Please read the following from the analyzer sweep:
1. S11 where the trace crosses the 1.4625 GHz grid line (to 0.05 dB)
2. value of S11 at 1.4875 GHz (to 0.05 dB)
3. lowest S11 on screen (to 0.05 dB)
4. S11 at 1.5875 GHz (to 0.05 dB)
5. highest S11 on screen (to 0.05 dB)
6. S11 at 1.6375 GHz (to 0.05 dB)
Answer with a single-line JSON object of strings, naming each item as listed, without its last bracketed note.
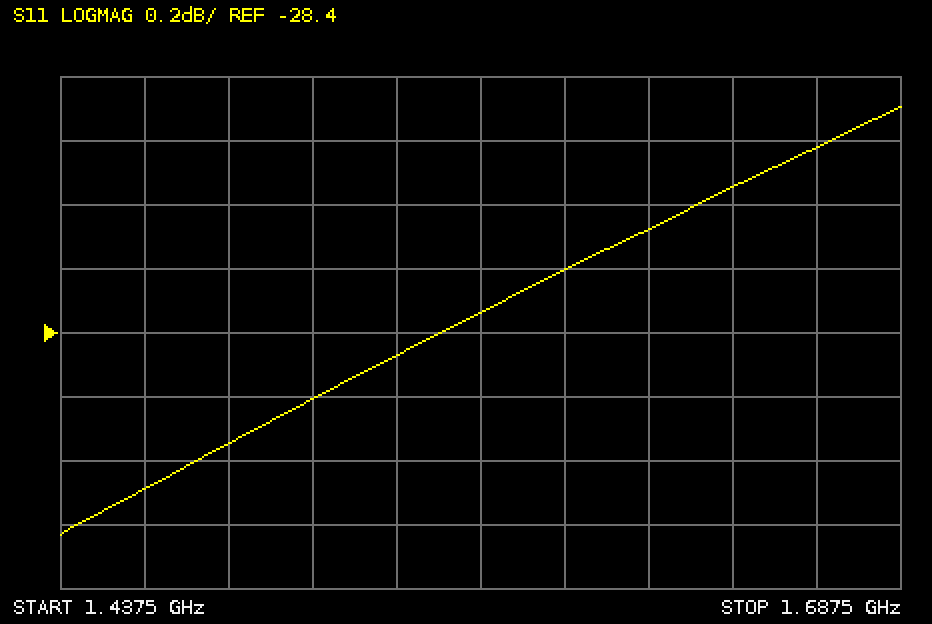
{"S11 where the trace crosses the 1.4625 GHz grid line": "-28.90 dB", "value of S11 at 1.4875 GHz": "-28.75 dB", "lowest S11 on screen": "-29.05 dB", "S11 at 1.5875 GHz": "-28.20 dB", "highest S11 on screen": "-27.70 dB", "S11 at 1.6375 GHz": "-27.95 dB"}
